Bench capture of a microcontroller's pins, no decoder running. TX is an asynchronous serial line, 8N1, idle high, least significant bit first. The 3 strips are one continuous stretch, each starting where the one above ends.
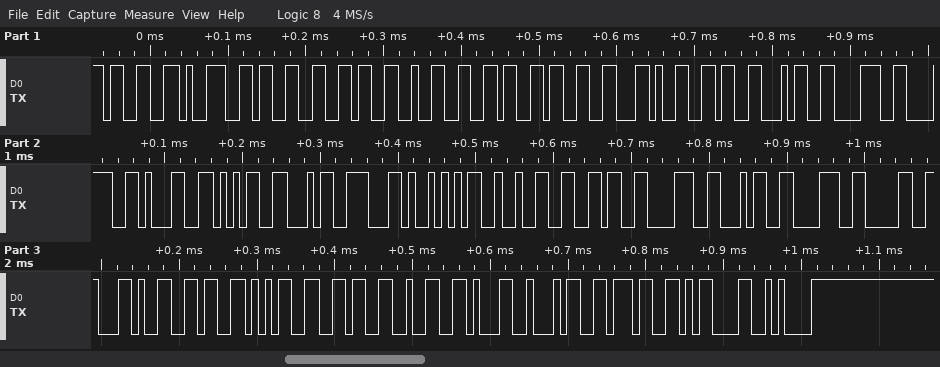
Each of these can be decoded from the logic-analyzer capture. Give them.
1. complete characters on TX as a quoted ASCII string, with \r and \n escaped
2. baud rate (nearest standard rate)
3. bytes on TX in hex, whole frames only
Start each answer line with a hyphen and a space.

- "3936263,6488154,5268480,6562147\r\n"
- 115200 baud
- 33 39 33 36 32 36 33 2C 36 34 38 38 31 35 34 2C 35 32 36 38 34 38 30 2C 36 35 36 32 31 34 37 0D 0A
